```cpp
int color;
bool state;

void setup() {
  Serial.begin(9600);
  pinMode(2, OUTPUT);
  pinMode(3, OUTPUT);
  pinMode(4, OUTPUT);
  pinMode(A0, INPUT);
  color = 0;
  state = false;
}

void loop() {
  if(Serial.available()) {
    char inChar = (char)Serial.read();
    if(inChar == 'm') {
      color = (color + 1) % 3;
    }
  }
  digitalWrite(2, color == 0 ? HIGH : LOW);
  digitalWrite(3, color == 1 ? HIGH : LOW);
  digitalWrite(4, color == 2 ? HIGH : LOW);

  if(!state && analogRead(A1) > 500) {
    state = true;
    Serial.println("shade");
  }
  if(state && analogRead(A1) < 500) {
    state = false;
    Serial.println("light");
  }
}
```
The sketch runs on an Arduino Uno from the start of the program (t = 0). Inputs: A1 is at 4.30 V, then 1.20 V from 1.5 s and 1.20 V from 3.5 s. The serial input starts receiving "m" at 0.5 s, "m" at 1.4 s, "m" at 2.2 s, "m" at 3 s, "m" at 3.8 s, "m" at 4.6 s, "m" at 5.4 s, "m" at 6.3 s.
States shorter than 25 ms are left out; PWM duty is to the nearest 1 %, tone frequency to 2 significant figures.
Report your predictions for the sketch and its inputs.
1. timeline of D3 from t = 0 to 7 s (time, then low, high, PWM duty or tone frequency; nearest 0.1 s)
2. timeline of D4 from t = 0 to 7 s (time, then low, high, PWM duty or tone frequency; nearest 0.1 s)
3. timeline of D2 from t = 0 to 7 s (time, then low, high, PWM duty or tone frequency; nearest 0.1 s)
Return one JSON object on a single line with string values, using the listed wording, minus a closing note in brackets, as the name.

{"timeline of D3 from t = 0 to 7 s": "0 s low; 0.5 s high; 1.4 s low; 3 s high; 3.8 s low; 5.4 s high; 6.3 s low", "timeline of D4 from t = 0 to 7 s": "0 s low; 1.4 s high; 2.2 s low; 3.8 s high; 4.6 s low; 6.3 s high", "timeline of D2 from t = 0 to 7 s": "0 s high; 0.5 s low; 2.2 s high; 3 s low; 4.6 s high; 5.4 s low"}
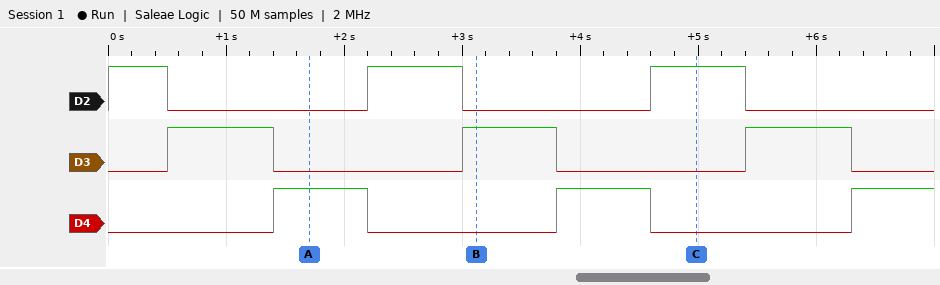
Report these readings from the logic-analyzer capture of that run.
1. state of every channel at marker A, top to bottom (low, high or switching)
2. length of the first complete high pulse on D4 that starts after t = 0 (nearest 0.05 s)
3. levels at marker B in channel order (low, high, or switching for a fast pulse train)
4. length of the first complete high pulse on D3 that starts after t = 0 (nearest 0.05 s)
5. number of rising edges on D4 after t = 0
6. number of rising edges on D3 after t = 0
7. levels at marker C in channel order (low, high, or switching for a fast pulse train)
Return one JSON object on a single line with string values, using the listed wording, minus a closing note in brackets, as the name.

{"state of every channel at marker A, top to bottom": "D2 low, D3 low, D4 high", "length of the first complete high pulse on D4 that starts after t = 0": "0.80 s", "levels at marker B in channel order": "D2 low, D3 high, D4 low", "length of the first complete high pulse on D3 that starts after t = 0": "0.90 s", "number of rising edges on D4 after t = 0": "3", "number of rising edges on D3 after t = 0": "3", "levels at marker C in channel order": "D2 high, D3 low, D4 low"}
